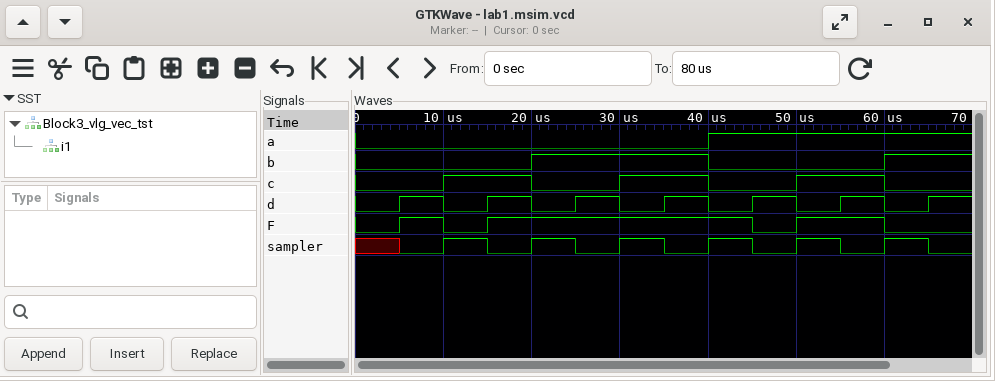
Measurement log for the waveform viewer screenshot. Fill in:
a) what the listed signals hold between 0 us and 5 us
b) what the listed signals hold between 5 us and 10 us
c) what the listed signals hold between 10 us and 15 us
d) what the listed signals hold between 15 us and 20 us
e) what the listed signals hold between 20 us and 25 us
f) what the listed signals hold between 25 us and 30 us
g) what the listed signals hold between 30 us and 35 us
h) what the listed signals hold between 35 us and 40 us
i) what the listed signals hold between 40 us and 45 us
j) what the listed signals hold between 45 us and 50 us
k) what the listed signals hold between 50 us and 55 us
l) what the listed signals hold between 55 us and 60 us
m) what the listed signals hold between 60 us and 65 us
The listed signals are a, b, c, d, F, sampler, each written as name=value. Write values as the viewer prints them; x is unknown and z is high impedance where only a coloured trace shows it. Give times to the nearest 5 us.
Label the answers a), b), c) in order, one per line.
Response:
a) a=0, b=0, c=0, d=0, F=0, sampler=x
b) a=0, b=0, c=0, d=1, F=1, sampler=0
c) a=0, b=0, c=1, d=0, F=0, sampler=1
d) a=0, b=0, c=1, d=1, F=1, sampler=0
e) a=0, b=1, c=0, d=0, F=1, sampler=1
f) a=0, b=1, c=0, d=1, F=1, sampler=0
g) a=0, b=1, c=1, d=0, F=1, sampler=1
h) a=0, b=1, c=1, d=1, F=1, sampler=0
i) a=1, b=0, c=0, d=0, F=1, sampler=1
j) a=1, b=0, c=0, d=1, F=0, sampler=0
k) a=1, b=0, c=1, d=0, F=1, sampler=1
l) a=1, b=0, c=1, d=1, F=1, sampler=0
m) a=1, b=1, c=0, d=0, F=0, sampler=1
